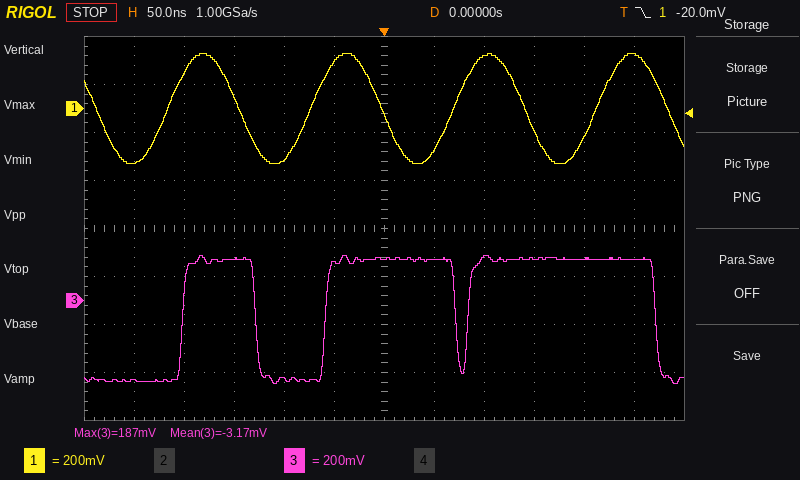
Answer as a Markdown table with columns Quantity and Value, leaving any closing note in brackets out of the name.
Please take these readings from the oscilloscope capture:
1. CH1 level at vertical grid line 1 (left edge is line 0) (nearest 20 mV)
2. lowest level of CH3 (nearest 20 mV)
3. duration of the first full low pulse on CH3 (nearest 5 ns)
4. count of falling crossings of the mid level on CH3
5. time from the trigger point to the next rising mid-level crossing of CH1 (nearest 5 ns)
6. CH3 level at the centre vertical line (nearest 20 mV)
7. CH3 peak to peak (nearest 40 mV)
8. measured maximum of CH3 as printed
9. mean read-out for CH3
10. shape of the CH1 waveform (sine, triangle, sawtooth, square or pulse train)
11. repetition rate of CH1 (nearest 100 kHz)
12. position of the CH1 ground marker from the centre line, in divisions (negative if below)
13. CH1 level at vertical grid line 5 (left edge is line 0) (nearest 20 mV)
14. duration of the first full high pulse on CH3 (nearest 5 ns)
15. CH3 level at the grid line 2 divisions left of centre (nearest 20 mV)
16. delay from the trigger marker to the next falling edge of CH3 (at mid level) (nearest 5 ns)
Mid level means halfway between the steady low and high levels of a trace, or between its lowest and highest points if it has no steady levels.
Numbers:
| Quantity | Value |
|---|---|
| CH1 level at vertical grid line 1 (left edge is line 0) | -220 mV |
| lowest level of CH3 | -340 mV |
| duration of the first full low pulse on CH3 | 70 ns |
| count of falling crossings of the mid level on CH3 | 3 |
| time from the trigger point to the next rising mid-level crossing of CH1 | 70 ns |
| CH3 level at the centre vertical line | 180 mV |
| CH3 peak to peak | 520 mV |
| measured maximum of CH3 as printed | 187 mV |
| mean read-out for CH3 | -3.17 mV |
| shape of the CH1 waveform | sine |
| repetition rate of CH1 | 7.0 MHz |
| position of the CH1 ground marker from the centre line, in divisions | +2.5 div |
| CH1 level at vertical grid line 5 (left edge is line 0) | 200 mV |
| duration of the first full high pulse on CH3 | 75 ns |
| CH3 level at the grid line 2 divisions left of centre | -320 mV |
| delay from the trigger marker to the next falling edge of CH3 (at mid level) | 70 ns |
